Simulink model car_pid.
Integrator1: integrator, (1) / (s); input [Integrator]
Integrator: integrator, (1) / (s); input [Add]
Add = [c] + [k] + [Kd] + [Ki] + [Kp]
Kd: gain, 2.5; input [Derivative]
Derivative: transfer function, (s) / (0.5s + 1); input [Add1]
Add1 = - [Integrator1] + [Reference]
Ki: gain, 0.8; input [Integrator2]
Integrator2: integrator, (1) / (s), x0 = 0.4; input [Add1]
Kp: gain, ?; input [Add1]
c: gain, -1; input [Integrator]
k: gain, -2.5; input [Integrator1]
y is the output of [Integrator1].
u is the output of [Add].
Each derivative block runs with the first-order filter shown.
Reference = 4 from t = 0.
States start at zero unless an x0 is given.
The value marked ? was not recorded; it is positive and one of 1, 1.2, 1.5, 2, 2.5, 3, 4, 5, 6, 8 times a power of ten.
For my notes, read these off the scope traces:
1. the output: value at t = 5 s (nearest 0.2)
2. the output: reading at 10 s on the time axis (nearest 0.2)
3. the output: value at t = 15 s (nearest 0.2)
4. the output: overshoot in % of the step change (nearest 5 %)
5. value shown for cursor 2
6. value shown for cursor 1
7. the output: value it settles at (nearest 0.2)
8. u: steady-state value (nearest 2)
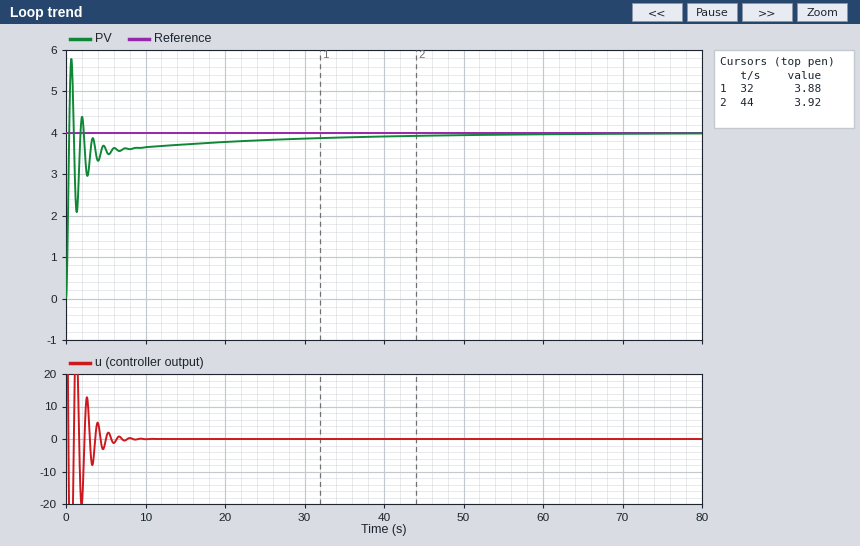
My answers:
3.6
3.6
3.8
45 %
3.92
3.88
4.0
0
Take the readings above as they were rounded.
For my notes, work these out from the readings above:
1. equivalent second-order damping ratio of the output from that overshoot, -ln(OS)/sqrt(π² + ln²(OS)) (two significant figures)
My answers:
0.25
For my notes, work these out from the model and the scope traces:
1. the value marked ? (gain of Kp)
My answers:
15
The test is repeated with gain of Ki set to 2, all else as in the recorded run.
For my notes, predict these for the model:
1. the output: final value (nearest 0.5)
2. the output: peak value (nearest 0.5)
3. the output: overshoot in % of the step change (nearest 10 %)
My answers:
4.0
6.0
50 %
